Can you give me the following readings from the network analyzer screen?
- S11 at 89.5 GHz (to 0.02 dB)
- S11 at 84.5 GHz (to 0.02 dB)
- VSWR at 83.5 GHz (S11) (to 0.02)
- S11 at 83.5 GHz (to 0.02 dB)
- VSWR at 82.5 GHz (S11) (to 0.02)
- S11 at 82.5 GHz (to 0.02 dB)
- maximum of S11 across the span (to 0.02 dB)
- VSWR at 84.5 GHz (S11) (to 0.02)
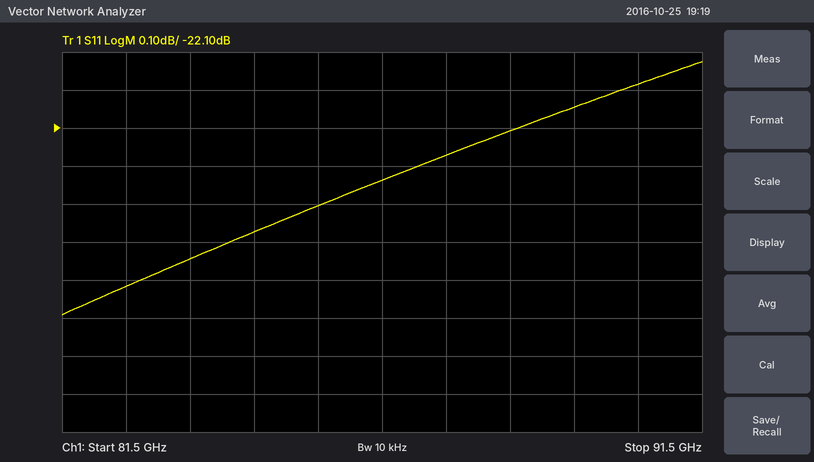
-22.04 dB
-22.38 dB
1.16
-22.44 dB
1.16
-22.52 dB
-21.92 dB
1.16
